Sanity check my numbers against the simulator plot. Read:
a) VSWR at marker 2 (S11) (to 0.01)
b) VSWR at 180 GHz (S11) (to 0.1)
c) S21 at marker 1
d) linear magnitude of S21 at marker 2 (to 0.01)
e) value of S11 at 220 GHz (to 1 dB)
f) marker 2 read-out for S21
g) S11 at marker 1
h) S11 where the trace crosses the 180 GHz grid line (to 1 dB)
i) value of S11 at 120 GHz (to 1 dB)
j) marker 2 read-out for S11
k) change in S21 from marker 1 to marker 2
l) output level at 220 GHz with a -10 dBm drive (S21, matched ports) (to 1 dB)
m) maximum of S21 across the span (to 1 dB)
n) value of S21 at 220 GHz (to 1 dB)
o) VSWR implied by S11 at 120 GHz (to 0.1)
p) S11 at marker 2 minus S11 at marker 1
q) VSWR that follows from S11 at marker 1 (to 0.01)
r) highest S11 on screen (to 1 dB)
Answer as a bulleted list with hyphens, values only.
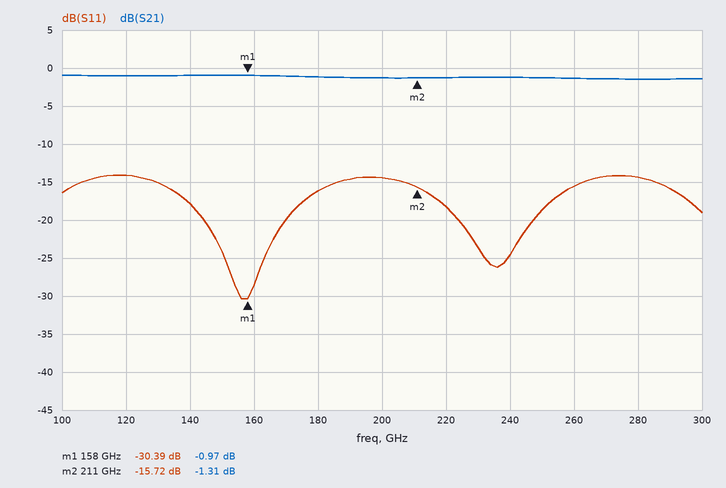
- 1.39
- 1.4
- -0.97 dB
- 0.86
- -18 dB
- -1.31 dB
- -30.39 dB
- -16 dB
- -14 dB
- -15.72 dB
- -0.34 dB
- -11 dBm
- -1 dB
- -1 dB
- 1.5
- 14.67 dB
- 1.06
- -14 dB
